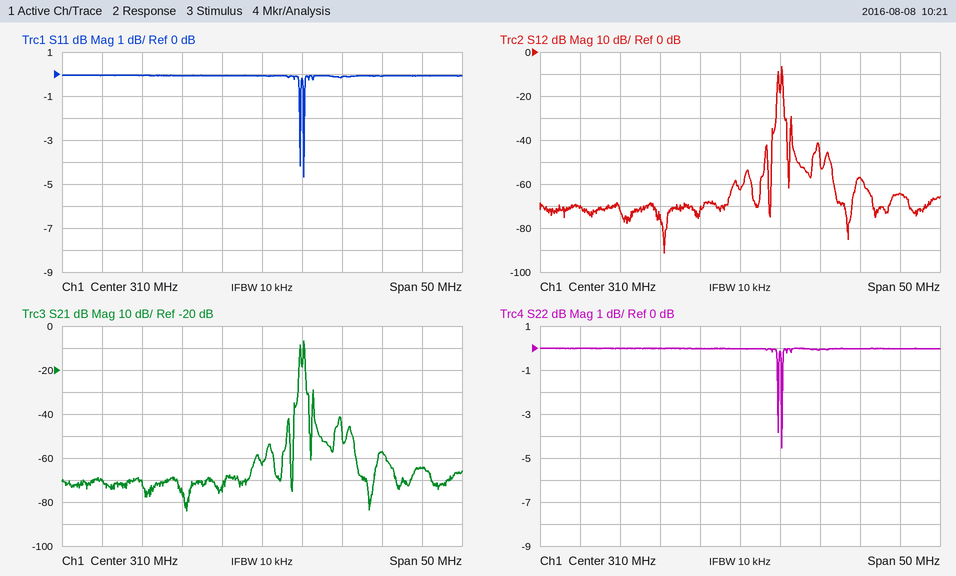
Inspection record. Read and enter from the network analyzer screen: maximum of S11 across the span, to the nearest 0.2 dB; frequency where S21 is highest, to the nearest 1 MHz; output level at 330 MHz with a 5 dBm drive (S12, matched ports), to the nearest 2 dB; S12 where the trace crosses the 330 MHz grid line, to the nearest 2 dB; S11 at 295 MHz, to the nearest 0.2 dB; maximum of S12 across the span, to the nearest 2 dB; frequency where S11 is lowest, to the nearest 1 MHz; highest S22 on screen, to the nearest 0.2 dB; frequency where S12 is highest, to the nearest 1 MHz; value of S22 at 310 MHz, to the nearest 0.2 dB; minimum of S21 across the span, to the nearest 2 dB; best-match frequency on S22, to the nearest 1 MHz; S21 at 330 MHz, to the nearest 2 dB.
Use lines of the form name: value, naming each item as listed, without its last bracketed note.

maximum of S11 across the span, to the nearest 0.2 dB: 0.0 dB
frequency where S21 is highest, to the nearest 1 MHz: 315 MHz
output level at 330 MHz with a 5 dBm drive (S12, matched ports), to the nearest 2 dB: -60 dBm
S12 where the trace crosses the 330 MHz grid line, to the nearest 2 dB: -64 dB
S11 at 295 MHz, to the nearest 0.2 dB: 0.0 dB
maximum of S12 across the span, to the nearest 2 dB: -6 dB
frequency where S11 is lowest, to the nearest 1 MHz: 315 MHz
highest S22 on screen, to the nearest 0.2 dB: 0.0 dB
frequency where S12 is highest, to the nearest 1 MHz: 315 MHz
value of S22 at 310 MHz, to the nearest 0.2 dB: 0.0 dB
minimum of S21 across the span, to the nearest 2 dB: -84 dB
best-match frequency on S22, to the nearest 1 MHz: 315 MHz
S21 at 330 MHz, to the nearest 2 dB: -64 dB
